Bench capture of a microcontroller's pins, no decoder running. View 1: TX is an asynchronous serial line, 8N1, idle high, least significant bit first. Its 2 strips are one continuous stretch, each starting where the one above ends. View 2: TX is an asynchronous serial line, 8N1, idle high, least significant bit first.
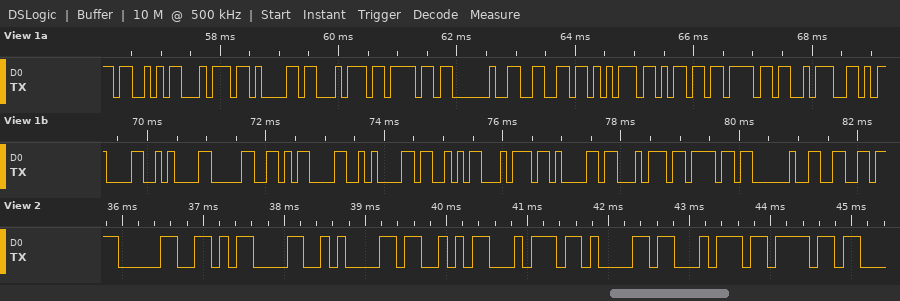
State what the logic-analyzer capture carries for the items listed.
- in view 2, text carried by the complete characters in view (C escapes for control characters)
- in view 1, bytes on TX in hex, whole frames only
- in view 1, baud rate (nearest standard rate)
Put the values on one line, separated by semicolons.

"0\r\nStato"; 53 74 61 74 6F 20 66 75 6D 6F 3A 0D 0A 30 0D 0A 53 74 61 74 6F 20 66; 9600 baud
